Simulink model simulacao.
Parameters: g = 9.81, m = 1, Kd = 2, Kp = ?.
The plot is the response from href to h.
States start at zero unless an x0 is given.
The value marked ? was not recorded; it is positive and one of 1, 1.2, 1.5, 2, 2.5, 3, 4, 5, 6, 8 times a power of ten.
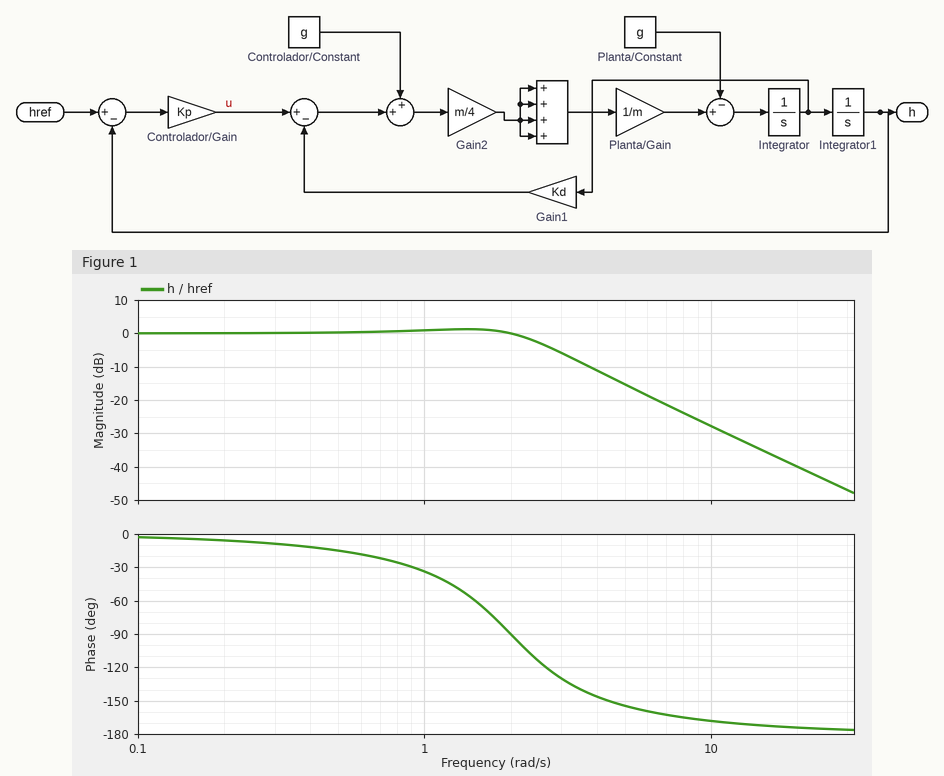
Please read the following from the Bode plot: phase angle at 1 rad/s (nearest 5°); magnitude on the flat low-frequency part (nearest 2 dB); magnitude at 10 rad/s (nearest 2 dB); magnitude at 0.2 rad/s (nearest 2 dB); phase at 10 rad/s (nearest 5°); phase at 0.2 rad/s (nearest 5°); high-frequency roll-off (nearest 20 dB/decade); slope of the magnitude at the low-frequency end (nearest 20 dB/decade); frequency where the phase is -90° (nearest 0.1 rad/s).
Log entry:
-35°
0 dB
-28 dB
0 dB
-170°
-5°
-40 dB/decade
0 dB/decade
2.0 rad/s
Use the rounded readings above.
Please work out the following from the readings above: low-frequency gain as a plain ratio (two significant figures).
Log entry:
1.0
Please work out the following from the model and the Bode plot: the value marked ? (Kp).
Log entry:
4
